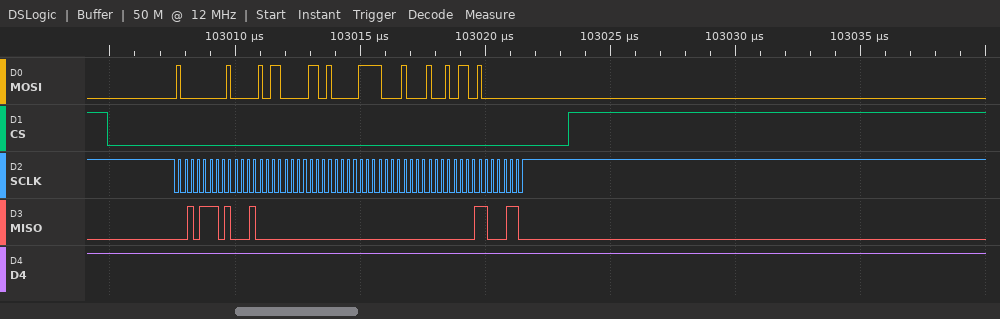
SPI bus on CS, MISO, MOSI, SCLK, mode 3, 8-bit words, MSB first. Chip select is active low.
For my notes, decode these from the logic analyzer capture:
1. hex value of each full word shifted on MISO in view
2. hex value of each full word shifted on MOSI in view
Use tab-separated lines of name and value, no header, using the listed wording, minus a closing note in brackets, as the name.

hex value of each full word shifted on MISO in view	2E, 88, 00, 00, 00, 00, C6
hex value of each full word shifted on MOSI in view	80, 85, 86, 87, 88, 96, 80
